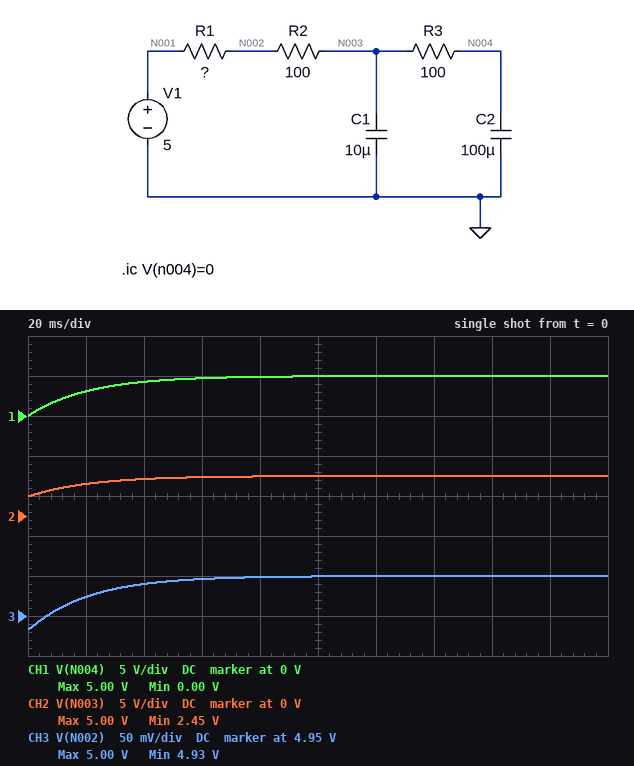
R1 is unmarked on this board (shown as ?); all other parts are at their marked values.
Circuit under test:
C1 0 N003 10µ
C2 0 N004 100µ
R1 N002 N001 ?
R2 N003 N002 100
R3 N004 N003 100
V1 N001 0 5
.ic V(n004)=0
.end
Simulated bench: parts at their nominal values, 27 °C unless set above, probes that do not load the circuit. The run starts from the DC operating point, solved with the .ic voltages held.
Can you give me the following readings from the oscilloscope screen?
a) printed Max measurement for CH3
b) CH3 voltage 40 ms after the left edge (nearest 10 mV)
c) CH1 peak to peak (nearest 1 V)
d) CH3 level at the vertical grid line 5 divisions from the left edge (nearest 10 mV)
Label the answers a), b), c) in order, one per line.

a) 5.00 V
b) 4.99 V
c) 5 V
d) 5.00 V
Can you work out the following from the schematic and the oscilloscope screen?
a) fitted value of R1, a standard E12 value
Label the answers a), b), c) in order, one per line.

a) 2.7 Ω
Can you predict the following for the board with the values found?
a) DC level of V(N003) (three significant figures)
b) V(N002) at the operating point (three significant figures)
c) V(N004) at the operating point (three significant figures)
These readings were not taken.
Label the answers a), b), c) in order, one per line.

a) 5.00 V
b) 5.00 V
c) 5.00 V
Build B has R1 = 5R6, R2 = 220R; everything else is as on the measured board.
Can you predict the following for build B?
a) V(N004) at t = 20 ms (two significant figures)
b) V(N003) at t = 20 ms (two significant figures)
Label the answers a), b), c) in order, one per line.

a) 2.2 V
b) 3.0 V
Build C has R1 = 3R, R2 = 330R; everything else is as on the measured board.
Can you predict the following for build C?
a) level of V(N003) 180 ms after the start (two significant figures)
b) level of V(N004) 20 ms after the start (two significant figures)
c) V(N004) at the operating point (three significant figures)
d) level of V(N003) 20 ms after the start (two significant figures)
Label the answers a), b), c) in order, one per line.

a) 4.9 V
b) 1.8 V
c) 5.00 V
d) 2.5 V
